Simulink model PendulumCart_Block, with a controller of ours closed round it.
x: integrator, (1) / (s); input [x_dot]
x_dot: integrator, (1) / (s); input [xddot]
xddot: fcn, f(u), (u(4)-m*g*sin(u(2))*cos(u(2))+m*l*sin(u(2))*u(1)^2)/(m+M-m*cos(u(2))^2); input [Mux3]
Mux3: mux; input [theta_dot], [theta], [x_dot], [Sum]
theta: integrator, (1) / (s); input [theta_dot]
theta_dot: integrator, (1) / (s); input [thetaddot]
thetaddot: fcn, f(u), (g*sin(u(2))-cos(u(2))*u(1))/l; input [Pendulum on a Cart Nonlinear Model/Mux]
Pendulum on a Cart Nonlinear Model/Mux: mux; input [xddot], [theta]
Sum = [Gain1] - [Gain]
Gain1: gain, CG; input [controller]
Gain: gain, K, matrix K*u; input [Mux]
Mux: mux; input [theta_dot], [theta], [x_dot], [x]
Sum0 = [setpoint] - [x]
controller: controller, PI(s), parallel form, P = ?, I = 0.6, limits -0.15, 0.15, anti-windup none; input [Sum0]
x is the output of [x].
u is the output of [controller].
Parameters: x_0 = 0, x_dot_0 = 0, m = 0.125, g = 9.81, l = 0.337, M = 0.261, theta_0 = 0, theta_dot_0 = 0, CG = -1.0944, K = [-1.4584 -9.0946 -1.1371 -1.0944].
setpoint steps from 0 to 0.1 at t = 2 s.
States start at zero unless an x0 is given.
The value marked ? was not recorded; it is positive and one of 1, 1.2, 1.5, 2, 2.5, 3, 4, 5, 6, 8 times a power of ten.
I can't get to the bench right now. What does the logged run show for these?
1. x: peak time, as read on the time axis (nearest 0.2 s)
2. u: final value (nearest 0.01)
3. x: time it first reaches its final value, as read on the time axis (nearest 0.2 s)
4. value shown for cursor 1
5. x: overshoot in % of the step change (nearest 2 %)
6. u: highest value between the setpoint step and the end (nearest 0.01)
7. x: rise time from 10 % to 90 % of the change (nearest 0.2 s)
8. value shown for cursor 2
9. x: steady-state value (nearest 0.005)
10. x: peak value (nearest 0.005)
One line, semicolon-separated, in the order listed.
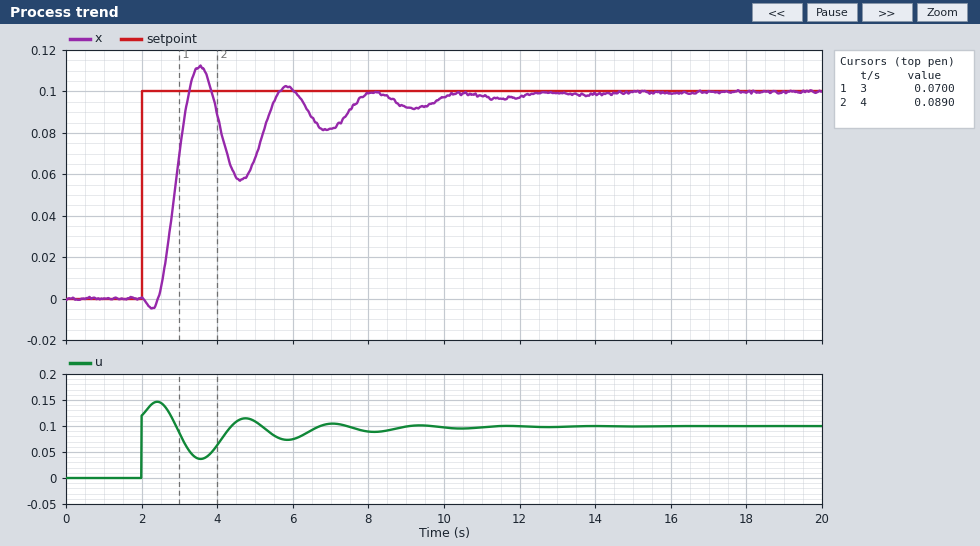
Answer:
3.6 s; 0.10; 3.2 s; 0.0700; 12 %; 0.15; 0.6 s; 0.0890; 0.100; 0.110
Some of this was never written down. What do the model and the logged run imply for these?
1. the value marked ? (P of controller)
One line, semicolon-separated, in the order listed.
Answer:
1.2
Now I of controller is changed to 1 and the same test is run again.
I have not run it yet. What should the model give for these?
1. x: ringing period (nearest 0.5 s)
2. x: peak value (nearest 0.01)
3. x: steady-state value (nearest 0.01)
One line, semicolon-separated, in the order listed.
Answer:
2.5 s; 0.13; 0.10
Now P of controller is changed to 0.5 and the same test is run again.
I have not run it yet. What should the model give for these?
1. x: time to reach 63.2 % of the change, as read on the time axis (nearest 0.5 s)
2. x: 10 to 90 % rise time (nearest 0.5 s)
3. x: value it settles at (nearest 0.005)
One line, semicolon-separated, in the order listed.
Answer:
3.5 s; 3.0 s; 0.100
